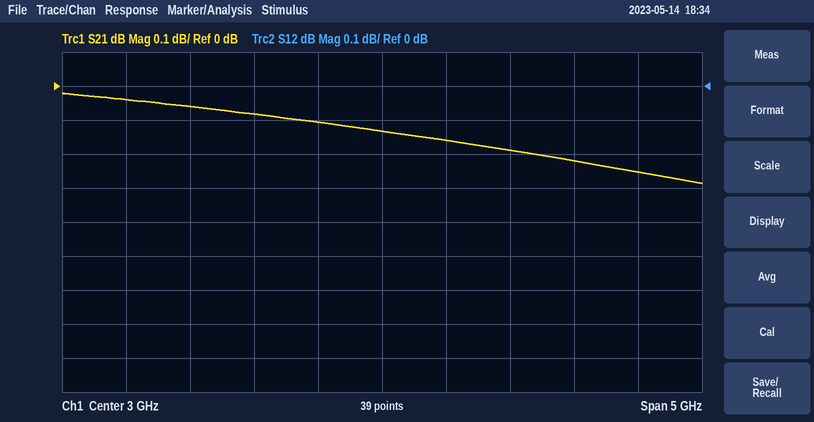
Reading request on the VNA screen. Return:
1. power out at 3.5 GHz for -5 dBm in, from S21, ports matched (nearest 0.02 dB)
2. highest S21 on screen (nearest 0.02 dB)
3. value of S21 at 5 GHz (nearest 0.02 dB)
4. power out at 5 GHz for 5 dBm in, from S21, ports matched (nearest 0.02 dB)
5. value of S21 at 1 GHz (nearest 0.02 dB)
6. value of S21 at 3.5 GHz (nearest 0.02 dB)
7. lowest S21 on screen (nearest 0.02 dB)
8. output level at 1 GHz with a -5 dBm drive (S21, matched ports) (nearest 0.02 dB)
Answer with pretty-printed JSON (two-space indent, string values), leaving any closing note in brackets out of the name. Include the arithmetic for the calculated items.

{
  "power out at 3.5 GHz for -5 dBm in, from S21, ports matched": "-5 dBm + (-0.16 dB) = -5.16 dBm",
  "highest S21 on screen": "-0.02 dB",
  "value of S21 at 5 GHz": "-0.26 dB",
  "power out at 5 GHz for 5 dBm in, from S21, ports matched": "5 dBm + (-0.26 dB) = 4.74 dBm",
  "value of S21 at 1 GHz": "-0.04 dB",
  "value of S21 at 3.5 GHz": "-0.16 dB",
  "lowest S21 on screen": "-0.28 dB",
  "output level at 1 GHz with a -5 dBm drive (S21, matched ports)": "-5 dBm + (-0.04 dB) = -5.04 dBm"
}
